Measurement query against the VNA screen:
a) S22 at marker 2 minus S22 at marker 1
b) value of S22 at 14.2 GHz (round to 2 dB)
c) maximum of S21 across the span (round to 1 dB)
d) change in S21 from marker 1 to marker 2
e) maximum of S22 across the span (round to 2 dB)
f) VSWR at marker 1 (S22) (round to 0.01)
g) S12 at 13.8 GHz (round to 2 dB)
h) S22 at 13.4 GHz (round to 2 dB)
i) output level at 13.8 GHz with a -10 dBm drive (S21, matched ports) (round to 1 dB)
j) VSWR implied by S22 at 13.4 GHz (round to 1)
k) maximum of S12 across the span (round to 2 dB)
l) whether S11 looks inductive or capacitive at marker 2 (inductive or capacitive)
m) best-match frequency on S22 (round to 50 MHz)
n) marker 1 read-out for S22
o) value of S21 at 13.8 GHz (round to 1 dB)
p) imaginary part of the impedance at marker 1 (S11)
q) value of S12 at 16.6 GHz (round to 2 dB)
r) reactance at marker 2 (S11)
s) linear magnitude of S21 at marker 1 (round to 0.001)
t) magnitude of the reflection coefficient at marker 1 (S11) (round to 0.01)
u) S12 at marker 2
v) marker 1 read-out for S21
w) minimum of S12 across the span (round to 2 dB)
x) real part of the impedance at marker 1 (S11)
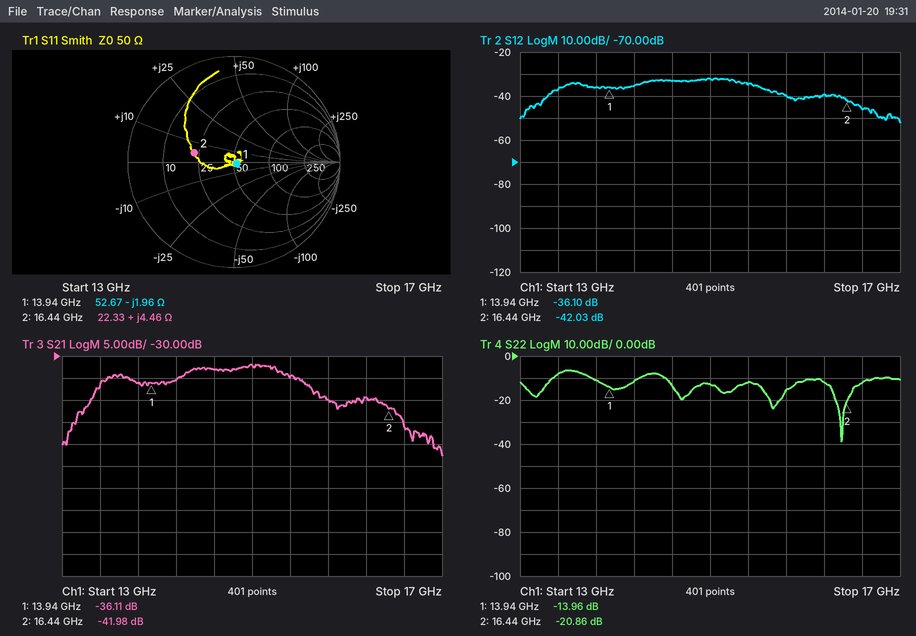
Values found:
-6.90 dB
-12 dB
-32 dB
-5.87 dB
-6 dB
1.50
-36 dB
-8 dB
-46 dBm
2
-32 dB
inductive
16.40 GHz
-13.96 dB
-36 dB
-1.96 Ω
-46 dB
+4.46 Ω
0.016
0.03
-42.03 dB
-36.11 dB
-52 dB
52.67 Ω
